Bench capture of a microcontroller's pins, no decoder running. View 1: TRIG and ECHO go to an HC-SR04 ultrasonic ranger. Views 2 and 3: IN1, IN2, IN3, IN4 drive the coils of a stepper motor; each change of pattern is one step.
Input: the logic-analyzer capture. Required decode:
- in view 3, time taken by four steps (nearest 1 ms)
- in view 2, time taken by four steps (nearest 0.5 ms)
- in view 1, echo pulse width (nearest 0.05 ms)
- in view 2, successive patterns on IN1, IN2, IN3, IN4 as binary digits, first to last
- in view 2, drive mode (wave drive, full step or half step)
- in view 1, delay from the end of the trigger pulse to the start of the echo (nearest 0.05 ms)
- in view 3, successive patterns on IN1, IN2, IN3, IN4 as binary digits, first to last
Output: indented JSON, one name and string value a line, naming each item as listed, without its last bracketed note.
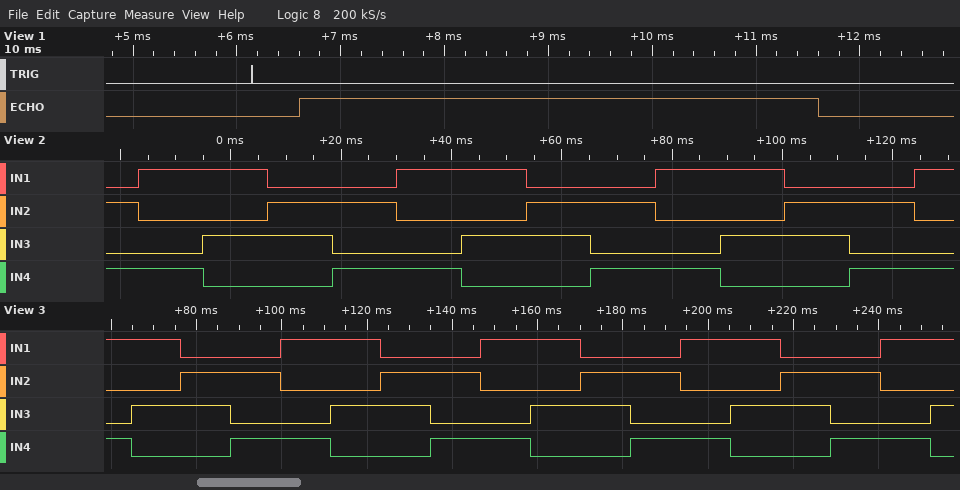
{
  "in view 3, time taken by four steps": "47 ms",
  "in view 2, time taken by four steps": "47.0 ms",
  "in view 1, echo pulse width": "5.00 ms",
  "in view 2, successive patterns on IN1, IN2, IN3, IN4 as binary digits, first to last": "0101 1001 1010 0110 0101 1001 1010 0110 0101 1001 1010 0110 0101 1001",
  "in view 2, drive mode": "full step",
  "in view 1, delay from the end of the trigger pulse to the start of the echo": "0.45 ms",
  "in view 3, successive patterns on IN1, IN2, IN3, IN4 as binary digits, first to last": "1001 1010 0110 0101 1001 1010 0110 0101 1001 1010 0110 0101 1001 1010 0110 0101 1001 1010"
}
